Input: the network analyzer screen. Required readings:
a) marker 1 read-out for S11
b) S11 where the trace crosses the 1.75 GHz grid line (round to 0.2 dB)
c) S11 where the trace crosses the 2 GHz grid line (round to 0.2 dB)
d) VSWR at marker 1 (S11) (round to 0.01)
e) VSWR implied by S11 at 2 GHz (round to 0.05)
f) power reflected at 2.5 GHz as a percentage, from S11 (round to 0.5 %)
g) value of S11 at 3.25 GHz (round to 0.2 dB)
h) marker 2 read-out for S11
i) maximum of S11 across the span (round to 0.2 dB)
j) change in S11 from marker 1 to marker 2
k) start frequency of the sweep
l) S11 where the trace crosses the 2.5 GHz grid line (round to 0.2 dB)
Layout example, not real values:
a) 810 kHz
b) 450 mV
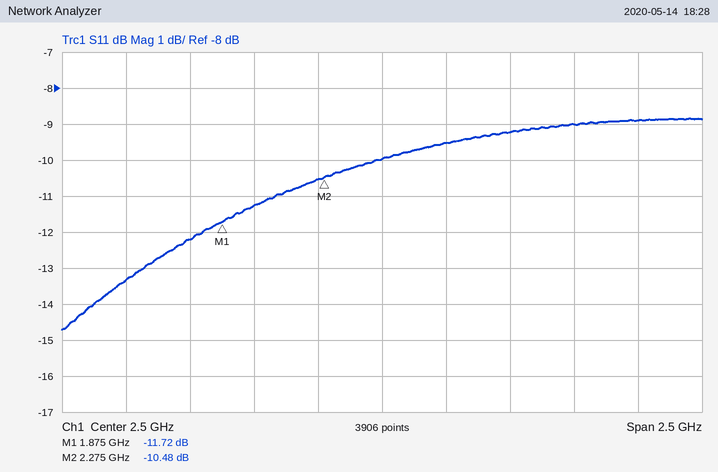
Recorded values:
a) -11.72 dB
b) -12.2 dB
c) -11.2 dB
d) 1.70
e) 1.75
f) 10.0 %
g) -9.0 dB
h) -10.48 dB
i) -8.8 dB
j) 1.24 dB
k) 1.25 GHz
l) -10.0 dB
